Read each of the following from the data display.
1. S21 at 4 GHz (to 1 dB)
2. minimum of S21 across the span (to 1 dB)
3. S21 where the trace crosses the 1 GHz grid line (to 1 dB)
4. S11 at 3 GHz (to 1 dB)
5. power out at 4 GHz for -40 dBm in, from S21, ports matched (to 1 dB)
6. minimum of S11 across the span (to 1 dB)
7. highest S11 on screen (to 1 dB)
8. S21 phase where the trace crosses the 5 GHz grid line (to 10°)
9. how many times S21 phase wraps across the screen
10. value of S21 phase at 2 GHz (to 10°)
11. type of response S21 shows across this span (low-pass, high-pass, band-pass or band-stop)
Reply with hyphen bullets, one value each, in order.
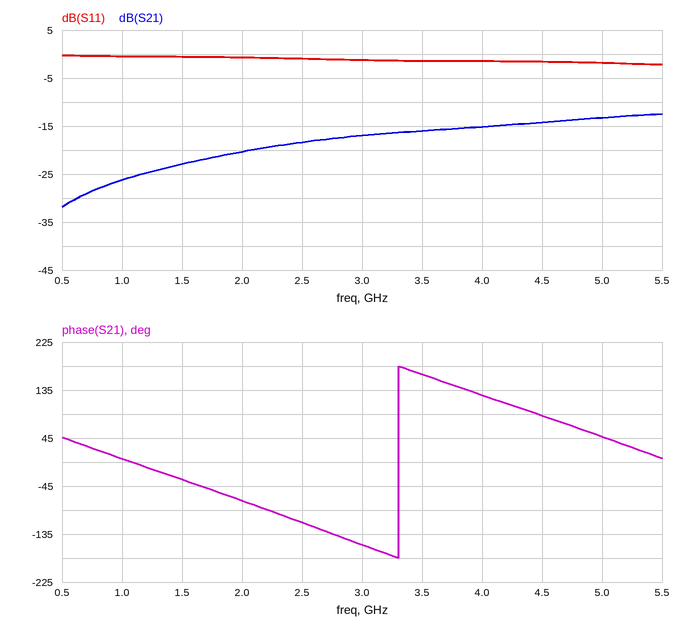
- -15 dB
- -32 dB
- -26 dB
- -1 dB
- -55 dBm
- -2 dB
- 0 dB
- 50°
- 1
- -70°
- high-pass
